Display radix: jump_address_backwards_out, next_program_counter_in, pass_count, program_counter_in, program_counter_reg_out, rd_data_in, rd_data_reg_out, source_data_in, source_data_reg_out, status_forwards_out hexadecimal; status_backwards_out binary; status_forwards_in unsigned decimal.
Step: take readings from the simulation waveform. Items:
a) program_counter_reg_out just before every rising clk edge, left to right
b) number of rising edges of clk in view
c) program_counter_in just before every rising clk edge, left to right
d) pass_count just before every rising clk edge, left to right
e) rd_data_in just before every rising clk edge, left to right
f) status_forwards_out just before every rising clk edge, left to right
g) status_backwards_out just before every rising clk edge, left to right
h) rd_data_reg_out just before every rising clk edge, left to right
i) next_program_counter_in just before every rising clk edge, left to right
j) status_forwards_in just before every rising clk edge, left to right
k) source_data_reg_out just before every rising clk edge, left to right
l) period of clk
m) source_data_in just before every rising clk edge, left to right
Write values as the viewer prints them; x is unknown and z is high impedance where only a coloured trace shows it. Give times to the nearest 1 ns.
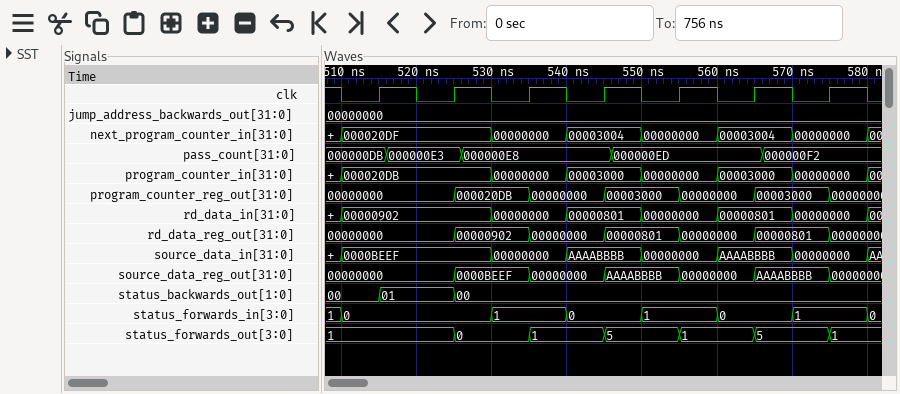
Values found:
00000000, 00000000, 000020DB, 00000000, 00003000, 00000000, 00003000
7
000020DB, 000020DB, 00000000, 00003000, 00000000, 00003000, 00000000
000000DB, 000000E3, 000000E8, 000000E8, 000000ED, 000000ED, 000000F2
00000902, 00000902, 00000000, 00000801, 00000000, 00000801, 00000000
1, 1, 0, 1, 5, 1, 5
00, 01, 00, 00, 00, 00, 00
00000000, 00000000, 00000902, 00000000, 00000801, 00000000, 00000801
000020DF, 000020DF, 00000000, 00003004, 00000000, 00003004, 00000000
0, 0, 1, 0, 1, 0, 1
00000000, 00000000, 0000BEEF, 00000000, AAAABBBB, 00000000, AAAABBBB
10 ns
0000BEEF, 0000BEEF, 00000000, AAAABBBB, 00000000, AAAABBBB, 00000000
